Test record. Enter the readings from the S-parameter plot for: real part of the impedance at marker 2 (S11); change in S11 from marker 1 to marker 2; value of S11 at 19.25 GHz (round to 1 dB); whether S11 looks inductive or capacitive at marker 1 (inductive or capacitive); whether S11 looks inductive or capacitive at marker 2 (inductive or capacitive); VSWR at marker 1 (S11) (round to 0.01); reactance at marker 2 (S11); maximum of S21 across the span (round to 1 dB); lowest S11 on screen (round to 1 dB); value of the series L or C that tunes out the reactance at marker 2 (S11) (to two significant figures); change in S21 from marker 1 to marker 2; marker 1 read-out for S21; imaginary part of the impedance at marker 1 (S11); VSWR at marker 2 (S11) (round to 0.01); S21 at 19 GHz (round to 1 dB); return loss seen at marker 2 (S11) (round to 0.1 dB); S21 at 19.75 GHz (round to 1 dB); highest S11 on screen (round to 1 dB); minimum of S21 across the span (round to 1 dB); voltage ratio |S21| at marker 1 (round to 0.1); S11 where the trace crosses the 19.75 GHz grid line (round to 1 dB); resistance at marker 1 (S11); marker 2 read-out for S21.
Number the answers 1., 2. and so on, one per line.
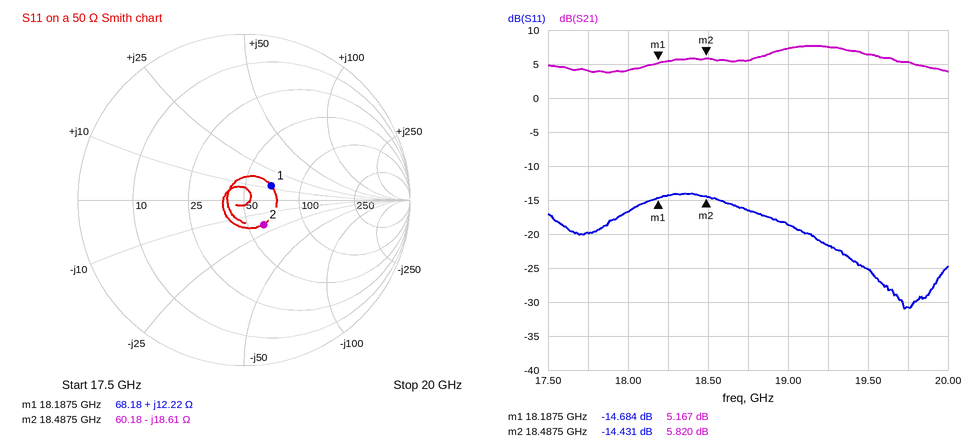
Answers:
1. 60.18 Ω
2. 0.253 dB
3. -22 dB
4. inductive
5. capacitive
6. 1.45
7. -18.61 Ω
8. 8 dB
9. -31 dB
10. 160 pH
11. 0.653 dB
12. 5.167 dB
13. +12.22 Ω
14. 1.47
15. 7 dB
16. 14.4 dB
17. 5 dB
18. -14 dB
19. 4 dB
20. 1.8
21. -31 dB
22. 68.18 Ω
23. 5.820 dB
